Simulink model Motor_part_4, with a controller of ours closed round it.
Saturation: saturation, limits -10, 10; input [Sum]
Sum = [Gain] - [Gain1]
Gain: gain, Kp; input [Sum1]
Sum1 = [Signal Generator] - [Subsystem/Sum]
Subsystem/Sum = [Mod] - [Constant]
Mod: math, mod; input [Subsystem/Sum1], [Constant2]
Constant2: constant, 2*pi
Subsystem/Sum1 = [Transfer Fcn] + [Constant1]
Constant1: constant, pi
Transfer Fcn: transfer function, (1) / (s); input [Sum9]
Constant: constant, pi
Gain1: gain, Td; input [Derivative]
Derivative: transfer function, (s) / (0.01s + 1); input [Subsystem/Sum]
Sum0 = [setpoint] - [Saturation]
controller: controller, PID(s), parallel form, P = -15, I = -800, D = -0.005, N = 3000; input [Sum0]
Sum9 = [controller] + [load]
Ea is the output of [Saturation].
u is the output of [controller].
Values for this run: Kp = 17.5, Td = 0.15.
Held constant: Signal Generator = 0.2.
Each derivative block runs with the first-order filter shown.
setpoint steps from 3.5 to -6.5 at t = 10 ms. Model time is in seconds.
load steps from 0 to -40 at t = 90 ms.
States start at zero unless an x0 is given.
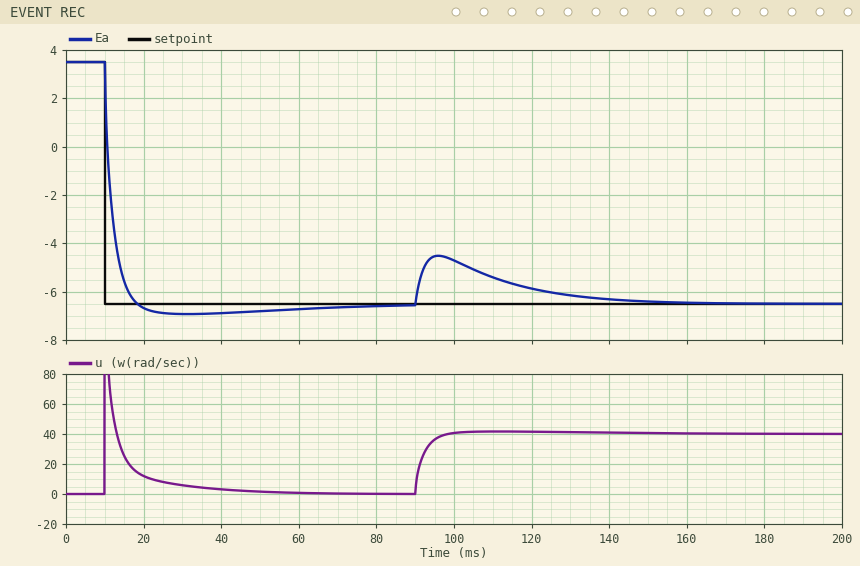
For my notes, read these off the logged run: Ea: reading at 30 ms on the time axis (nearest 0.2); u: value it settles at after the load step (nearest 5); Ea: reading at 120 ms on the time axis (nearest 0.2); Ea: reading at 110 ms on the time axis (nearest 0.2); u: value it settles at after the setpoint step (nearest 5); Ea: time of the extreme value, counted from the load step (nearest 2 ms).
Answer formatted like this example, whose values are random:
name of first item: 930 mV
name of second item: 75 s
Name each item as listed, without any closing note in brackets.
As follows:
Ea: reading at 30 ms on the time axis: -7.0
u: value it settles at after the load step: 40
Ea: reading at 120 ms on the time axis: -5.8
Ea: reading at 110 ms on the time axis: -5.4
u: value it settles at after the setpoint step: 0
Ea: time of the extreme value, counted from the load step: 6 ms
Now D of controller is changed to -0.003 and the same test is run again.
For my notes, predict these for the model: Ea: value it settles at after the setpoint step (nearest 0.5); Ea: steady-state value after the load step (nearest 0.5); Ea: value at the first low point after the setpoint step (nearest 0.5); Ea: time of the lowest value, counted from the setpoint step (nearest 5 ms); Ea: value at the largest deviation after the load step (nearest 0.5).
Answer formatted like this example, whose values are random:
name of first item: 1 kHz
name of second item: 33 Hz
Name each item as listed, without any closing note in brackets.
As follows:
Ea: value it settles at after the setpoint step: -6.5
Ea: steady-state value after the load step: -6.5
Ea: value at the first low point after the setpoint step: -7.0
Ea: time of the lowest value, counted from the setpoint step: 20 ms
Ea: value at the largest deviation after the load step: -4.5
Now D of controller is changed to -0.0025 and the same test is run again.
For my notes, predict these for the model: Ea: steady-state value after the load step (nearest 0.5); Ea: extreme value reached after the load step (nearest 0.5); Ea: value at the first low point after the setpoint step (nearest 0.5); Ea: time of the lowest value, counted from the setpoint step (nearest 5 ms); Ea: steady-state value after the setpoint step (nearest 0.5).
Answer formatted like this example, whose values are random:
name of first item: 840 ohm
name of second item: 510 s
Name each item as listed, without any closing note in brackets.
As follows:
Ea: steady-state value after the load step: -6.5
Ea: extreme value reached after the load step: -4.5
Ea: value at the first low point after the setpoint step: -7.0
Ea: time of the lowest value, counted from the setpoint step: 20 ms
Ea: steady-state value after the setpoint step: -6.5
